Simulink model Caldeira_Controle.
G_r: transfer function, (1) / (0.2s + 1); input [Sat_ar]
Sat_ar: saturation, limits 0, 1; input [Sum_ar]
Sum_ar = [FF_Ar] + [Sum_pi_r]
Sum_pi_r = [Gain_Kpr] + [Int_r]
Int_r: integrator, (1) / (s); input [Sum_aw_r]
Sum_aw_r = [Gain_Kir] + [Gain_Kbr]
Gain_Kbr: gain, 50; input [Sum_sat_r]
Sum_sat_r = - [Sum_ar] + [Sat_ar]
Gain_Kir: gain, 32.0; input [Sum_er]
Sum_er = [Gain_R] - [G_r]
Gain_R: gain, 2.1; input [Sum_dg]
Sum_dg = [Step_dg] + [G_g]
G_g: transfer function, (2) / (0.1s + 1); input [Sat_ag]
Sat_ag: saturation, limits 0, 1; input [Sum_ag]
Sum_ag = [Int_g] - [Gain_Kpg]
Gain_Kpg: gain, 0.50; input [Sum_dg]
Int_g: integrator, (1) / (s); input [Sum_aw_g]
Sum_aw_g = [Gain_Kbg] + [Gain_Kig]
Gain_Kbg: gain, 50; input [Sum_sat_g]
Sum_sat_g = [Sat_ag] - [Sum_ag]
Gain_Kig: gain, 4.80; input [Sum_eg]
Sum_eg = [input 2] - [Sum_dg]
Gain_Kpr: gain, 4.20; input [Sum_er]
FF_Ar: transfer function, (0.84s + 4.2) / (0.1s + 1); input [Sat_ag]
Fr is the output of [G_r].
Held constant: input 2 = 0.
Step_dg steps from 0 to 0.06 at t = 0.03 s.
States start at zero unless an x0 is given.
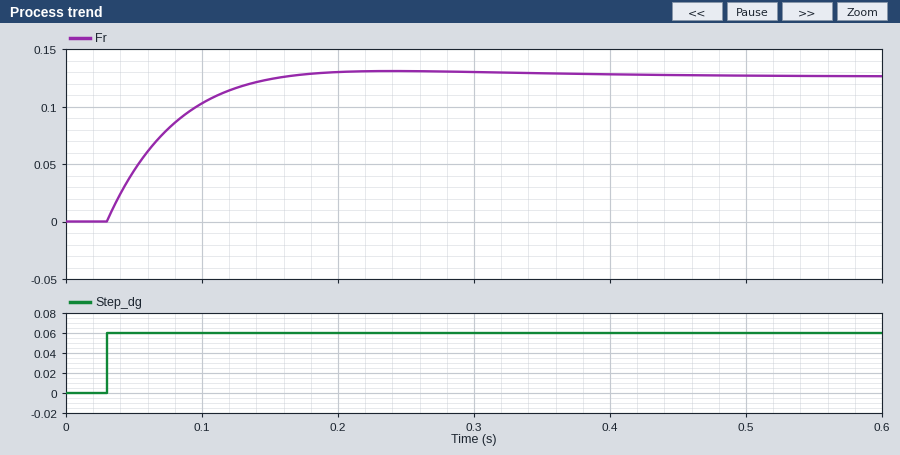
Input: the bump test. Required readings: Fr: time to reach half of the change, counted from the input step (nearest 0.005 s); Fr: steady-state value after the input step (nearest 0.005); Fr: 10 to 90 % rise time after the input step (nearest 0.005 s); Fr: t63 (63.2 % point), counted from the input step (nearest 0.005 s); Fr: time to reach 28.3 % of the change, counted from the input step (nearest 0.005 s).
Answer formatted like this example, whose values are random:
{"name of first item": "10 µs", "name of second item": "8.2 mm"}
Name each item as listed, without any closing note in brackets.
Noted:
{"Fr: time to reach half of the change, counted from the input step": "0.030 s", "Fr: steady-state value after the input step": "0.125", "Fr: 10 to 90 % rise time after the input step": "0.085 s", "Fr: t63 (63.2 % point), counted from the input step": "0.045 s", "Fr: time to reach 28.3 % of the change, counted from the input step": "0.015 s"}
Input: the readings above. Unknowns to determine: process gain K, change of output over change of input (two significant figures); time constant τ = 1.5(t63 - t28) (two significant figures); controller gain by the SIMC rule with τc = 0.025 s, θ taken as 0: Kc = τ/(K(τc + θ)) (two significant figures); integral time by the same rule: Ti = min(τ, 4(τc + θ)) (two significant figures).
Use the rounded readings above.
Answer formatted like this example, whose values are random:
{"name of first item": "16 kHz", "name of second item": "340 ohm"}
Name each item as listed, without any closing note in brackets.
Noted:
{"process gain K, change of output over change of input": "2.1", "time constant τ = 1.5(t63 - t28)": "0.045 s", "controller gain by the SIMC rule with τc = 0.025 s, θ taken as 0: Kc = τ/(K(τc + θ))": "0.86", "integral time by the same rule: Ti = min(τ, 4(τc + θ))": "0.045 s"}
